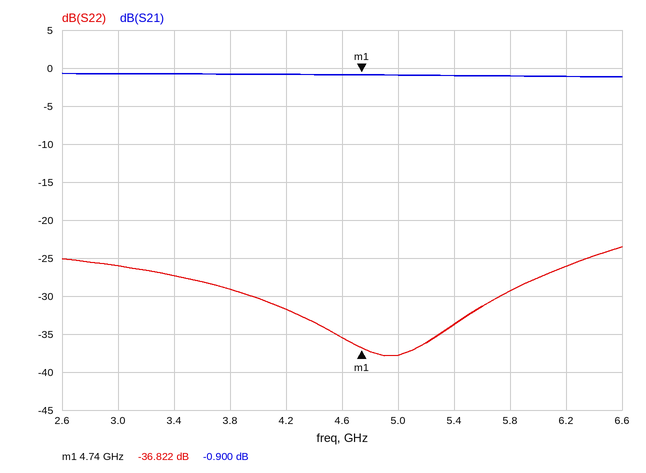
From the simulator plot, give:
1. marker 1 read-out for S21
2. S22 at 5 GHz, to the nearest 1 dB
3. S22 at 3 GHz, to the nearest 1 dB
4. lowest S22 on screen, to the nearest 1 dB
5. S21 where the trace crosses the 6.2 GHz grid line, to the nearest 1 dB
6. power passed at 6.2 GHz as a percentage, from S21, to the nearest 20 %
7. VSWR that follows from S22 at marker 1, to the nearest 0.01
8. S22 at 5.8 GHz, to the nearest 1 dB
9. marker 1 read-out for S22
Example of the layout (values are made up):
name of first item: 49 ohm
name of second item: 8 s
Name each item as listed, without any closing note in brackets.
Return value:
marker 1 read-out for S21: -0.900 dB
S22 at 5 GHz, to the nearest 1 dB: -38 dB
S22 at 3 GHz, to the nearest 1 dB: -26 dB
lowest S22 on screen, to the nearest 1 dB: -38 dB
S21 where the trace crosses the 6.2 GHz grid line, to the nearest 1 dB: -1 dB
power passed at 6.2 GHz as a percentage, from S21, to the nearest 20 %: 80 %
VSWR that follows from S22 at marker 1, to the nearest 0.01: 1.03
S22 at 5.8 GHz, to the nearest 1 dB: -29 dB
marker 1 read-out for S22: -36.822 dB
